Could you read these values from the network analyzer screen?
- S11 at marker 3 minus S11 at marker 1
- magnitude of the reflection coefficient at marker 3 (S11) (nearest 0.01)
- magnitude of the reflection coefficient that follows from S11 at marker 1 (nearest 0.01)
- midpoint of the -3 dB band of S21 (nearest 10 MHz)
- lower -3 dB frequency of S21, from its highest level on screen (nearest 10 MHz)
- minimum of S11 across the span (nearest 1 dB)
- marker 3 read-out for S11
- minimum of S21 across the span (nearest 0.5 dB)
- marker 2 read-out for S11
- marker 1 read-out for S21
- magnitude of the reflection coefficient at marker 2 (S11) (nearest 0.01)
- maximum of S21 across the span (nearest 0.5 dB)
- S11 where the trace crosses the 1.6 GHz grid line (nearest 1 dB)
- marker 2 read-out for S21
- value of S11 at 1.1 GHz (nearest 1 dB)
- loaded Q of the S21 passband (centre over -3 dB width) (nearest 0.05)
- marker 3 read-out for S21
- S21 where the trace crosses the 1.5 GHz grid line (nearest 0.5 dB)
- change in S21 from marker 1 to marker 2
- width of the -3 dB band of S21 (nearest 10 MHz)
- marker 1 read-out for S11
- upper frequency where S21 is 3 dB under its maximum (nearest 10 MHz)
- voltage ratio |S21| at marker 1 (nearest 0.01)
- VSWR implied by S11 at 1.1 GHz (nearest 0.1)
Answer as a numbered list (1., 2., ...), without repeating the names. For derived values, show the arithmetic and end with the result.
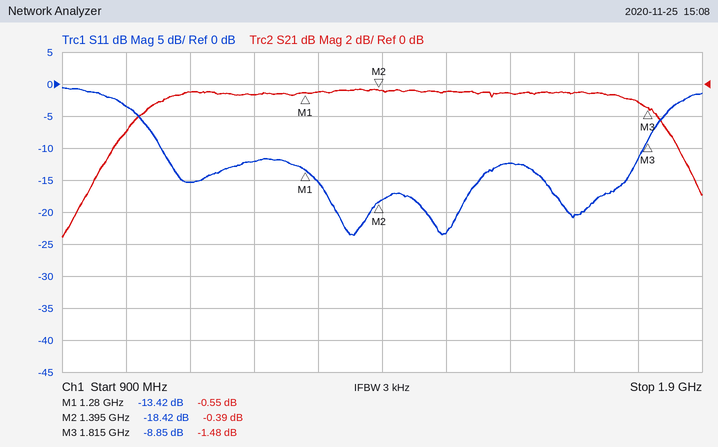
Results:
1. -8.85 − (-13.42) = 4.57 dB
2. 10^(-8.85/20) ≈ 0.36
3. 10^(-13.42/20) ≈ 0.21
4. 1.42 GHz
5. 990 MHz
6. -24 dB
7. -8.85 dB
8. -9.5 dB
9. -18.42 dB
10. -0.55 dB
11. 10^(-18.42/20) ≈ 0.12
12. -0.5 dB
13. -12 dB
14. -0.39 dB
15. -15 dB
16. 1.42 GHz / 860 MHz ≈ 1.65
17. -1.48 dB
18. -0.5 dB
19. -0.39 − (-0.55) = 0.16 dB
20. 1.85 GHz − 990 MHz = 860 MHz
21. -13.42 dB
22. 1.85 GHz
23. 10^(-0.55/20) ≈ 0.94
24. |Γ| = 10^(-15/20) = 0.1778; VSWR = (1 + 0.1778)/(1 − 0.1778) ≈ 1.4
